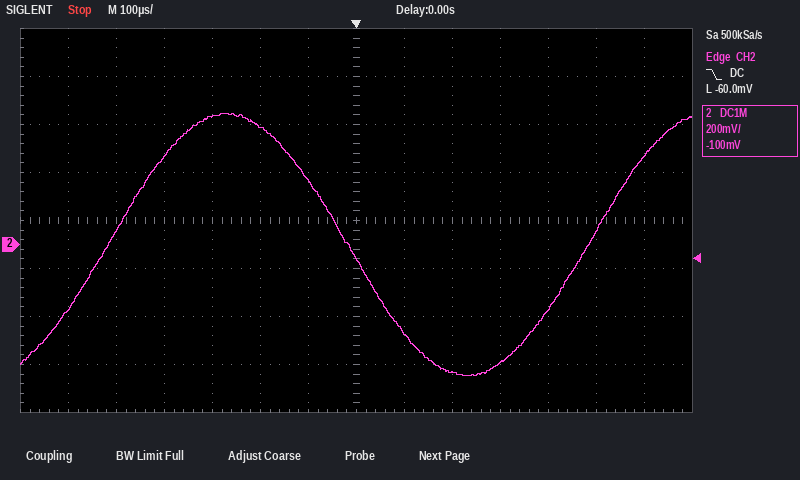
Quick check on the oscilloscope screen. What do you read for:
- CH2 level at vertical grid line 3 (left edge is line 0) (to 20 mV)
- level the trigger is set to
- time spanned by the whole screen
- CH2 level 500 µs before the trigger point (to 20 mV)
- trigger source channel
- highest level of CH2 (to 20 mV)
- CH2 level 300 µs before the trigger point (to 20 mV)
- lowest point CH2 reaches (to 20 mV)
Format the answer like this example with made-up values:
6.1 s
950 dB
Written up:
360 mV
-60.0 mV
1.4 ms
60 mV
CH2
540 mV
540 mV
-540 mV
